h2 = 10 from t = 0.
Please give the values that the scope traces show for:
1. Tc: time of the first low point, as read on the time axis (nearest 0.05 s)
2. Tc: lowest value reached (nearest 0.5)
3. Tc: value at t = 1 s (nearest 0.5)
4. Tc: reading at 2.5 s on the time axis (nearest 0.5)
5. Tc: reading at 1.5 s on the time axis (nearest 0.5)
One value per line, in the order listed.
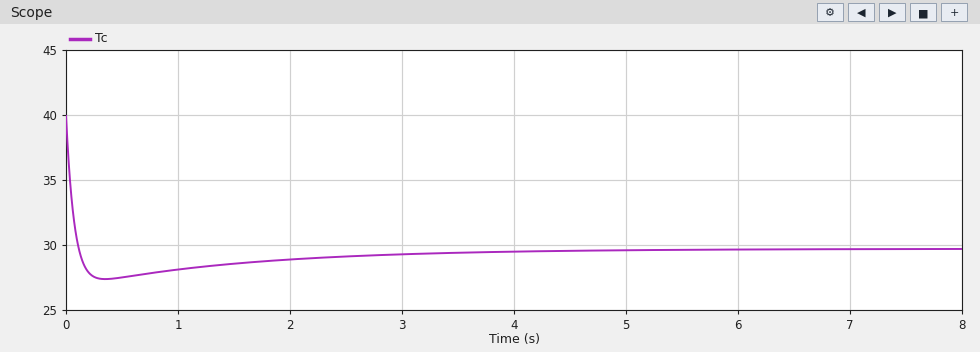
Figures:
0.35 s
27.5
28.0
29.0
28.5
